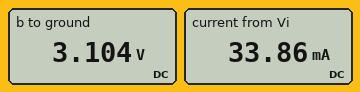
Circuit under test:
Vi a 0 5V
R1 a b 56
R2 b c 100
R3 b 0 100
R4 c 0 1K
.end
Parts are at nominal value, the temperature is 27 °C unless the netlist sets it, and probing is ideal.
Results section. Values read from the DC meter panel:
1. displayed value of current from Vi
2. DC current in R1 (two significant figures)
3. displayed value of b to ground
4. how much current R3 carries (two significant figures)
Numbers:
33.86 mA
34 mA
3.104 V
31 mA
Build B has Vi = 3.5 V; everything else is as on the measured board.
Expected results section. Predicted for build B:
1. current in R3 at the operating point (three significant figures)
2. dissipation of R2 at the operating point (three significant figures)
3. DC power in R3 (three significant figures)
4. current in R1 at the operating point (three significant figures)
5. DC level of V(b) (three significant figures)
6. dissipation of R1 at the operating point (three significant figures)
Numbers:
21.7 mA
390 µW
47.2 mW
23.7 mA
2.17 V
31.5 mW
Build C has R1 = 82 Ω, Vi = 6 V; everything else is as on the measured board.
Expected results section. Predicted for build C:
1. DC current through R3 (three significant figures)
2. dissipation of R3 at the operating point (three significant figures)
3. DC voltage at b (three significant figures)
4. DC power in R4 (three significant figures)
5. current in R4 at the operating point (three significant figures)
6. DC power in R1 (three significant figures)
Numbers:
31.7 mA
100 mW
3.17 V
8.29 mW
2.88 mA
97.9 mW
